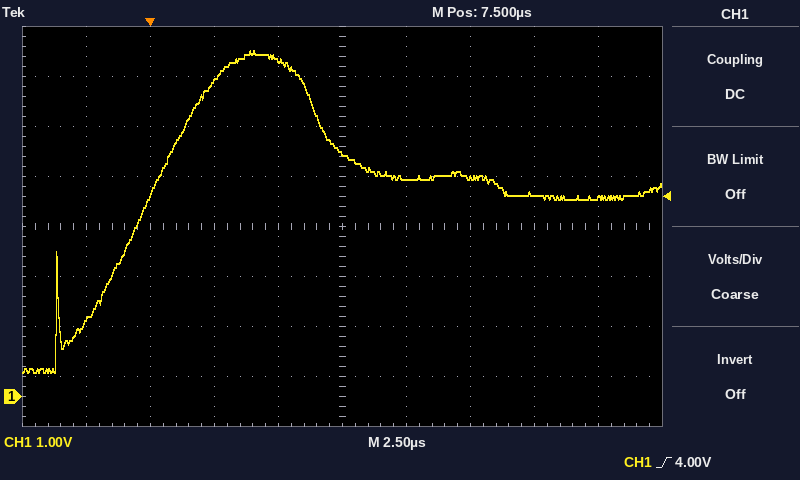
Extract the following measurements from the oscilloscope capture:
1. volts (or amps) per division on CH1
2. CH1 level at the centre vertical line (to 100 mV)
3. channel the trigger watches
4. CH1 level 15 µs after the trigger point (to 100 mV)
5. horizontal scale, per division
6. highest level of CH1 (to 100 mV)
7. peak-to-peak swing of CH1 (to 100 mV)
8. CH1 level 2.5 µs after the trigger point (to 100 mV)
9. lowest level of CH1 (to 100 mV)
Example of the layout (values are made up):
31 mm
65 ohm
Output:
1 V
4.9 V
CH1
4.0 V
2.5 µs
6.9 V
6.4 V
6.3 V
500 mV
